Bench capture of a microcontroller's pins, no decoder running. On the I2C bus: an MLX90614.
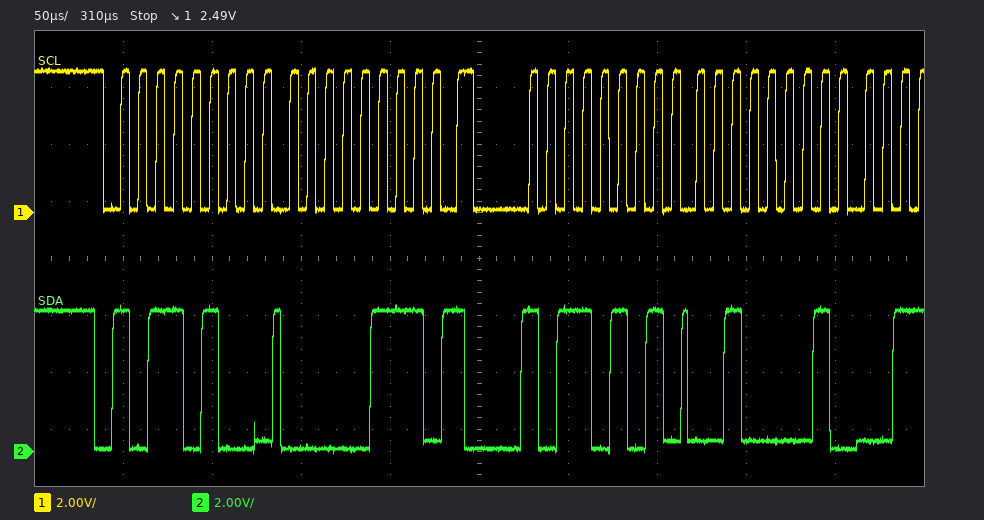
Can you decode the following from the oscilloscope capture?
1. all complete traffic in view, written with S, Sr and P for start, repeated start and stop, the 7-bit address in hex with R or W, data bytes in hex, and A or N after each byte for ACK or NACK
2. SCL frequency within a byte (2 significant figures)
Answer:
S 5AW A 07 A Sr 5AR A 21 A
100 kHz
